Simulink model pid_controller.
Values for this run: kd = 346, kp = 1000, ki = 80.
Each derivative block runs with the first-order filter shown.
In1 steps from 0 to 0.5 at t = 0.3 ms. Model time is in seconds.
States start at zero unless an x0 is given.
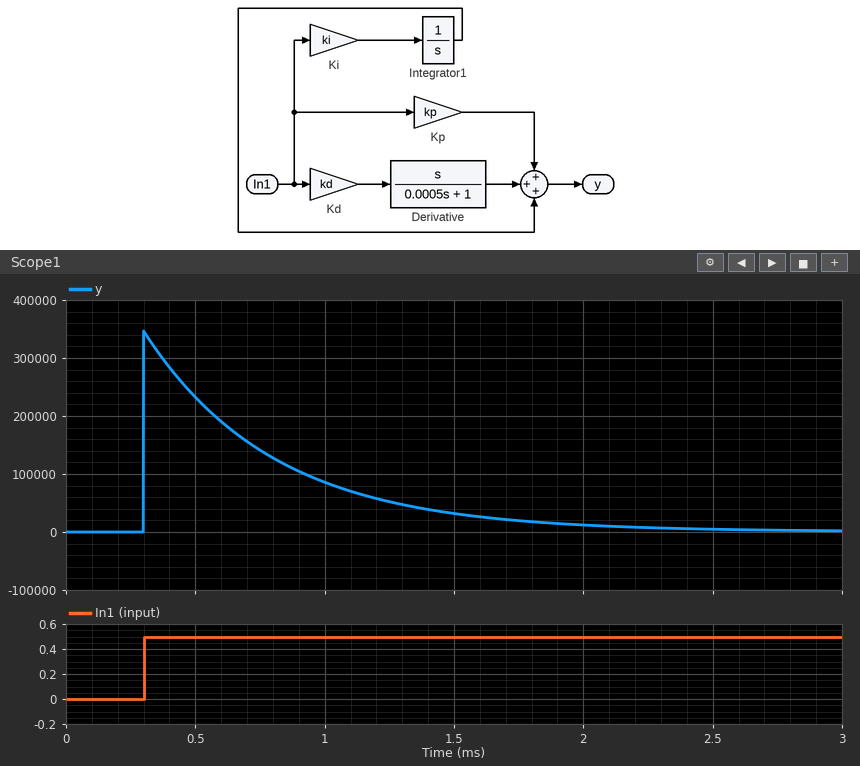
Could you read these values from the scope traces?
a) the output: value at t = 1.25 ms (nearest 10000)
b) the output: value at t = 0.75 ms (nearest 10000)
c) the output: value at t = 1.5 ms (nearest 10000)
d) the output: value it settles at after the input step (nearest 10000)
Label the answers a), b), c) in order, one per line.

a) 50000
b) 140000
c) 30000
d) 0
